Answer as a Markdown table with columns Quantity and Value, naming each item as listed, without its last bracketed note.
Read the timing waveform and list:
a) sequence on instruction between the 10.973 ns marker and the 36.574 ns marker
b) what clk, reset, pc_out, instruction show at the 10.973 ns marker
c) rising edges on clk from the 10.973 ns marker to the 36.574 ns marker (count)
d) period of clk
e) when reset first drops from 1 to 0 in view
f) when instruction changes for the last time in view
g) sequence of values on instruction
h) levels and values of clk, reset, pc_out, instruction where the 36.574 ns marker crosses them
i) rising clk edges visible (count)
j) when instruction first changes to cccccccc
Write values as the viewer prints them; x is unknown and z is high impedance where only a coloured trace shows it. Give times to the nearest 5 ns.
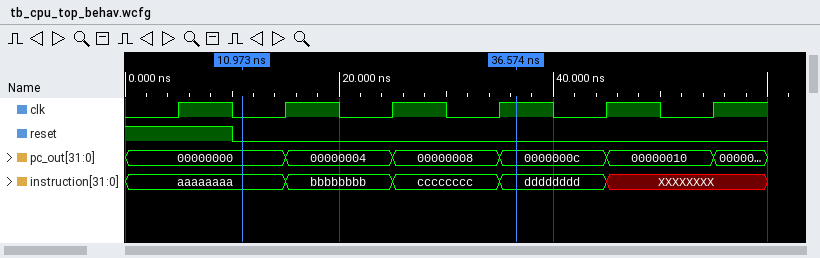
| Quantity | Value |
|---|---|
| sequence on instruction between the 10.973 ns marker and the 36.574 ns marker | aaaaaaaa, bbbbbbbb, cccccccc, dddddddd |
| what clk, reset, pc_out, instruction show at the 10.973 ns marker | clk=0, reset=0, pc_out=00000000, instruction=aaaaaaaa |
| rising edges on clk from the 10.973 ns marker to the 36.574 ns marker | 3 |
| period of clk | 10 ns |
| when reset first drops from 1 to 0 in view | 10 ns |
| when instruction changes for the last time in view | 45 ns |
| sequence of values on instruction | aaaaaaaa, bbbbbbbb, cccccccc, dddddddd, XXXXXXXX |
| levels and values of clk, reset, pc_out, instruction where the 36.574 ns marker crosses them | clk=1, reset=0, pc_out=0000000c, instruction=dddddddd |
| rising clk edges visible | 6 |
| when instruction first changes to cccccccc | 25 ns |
